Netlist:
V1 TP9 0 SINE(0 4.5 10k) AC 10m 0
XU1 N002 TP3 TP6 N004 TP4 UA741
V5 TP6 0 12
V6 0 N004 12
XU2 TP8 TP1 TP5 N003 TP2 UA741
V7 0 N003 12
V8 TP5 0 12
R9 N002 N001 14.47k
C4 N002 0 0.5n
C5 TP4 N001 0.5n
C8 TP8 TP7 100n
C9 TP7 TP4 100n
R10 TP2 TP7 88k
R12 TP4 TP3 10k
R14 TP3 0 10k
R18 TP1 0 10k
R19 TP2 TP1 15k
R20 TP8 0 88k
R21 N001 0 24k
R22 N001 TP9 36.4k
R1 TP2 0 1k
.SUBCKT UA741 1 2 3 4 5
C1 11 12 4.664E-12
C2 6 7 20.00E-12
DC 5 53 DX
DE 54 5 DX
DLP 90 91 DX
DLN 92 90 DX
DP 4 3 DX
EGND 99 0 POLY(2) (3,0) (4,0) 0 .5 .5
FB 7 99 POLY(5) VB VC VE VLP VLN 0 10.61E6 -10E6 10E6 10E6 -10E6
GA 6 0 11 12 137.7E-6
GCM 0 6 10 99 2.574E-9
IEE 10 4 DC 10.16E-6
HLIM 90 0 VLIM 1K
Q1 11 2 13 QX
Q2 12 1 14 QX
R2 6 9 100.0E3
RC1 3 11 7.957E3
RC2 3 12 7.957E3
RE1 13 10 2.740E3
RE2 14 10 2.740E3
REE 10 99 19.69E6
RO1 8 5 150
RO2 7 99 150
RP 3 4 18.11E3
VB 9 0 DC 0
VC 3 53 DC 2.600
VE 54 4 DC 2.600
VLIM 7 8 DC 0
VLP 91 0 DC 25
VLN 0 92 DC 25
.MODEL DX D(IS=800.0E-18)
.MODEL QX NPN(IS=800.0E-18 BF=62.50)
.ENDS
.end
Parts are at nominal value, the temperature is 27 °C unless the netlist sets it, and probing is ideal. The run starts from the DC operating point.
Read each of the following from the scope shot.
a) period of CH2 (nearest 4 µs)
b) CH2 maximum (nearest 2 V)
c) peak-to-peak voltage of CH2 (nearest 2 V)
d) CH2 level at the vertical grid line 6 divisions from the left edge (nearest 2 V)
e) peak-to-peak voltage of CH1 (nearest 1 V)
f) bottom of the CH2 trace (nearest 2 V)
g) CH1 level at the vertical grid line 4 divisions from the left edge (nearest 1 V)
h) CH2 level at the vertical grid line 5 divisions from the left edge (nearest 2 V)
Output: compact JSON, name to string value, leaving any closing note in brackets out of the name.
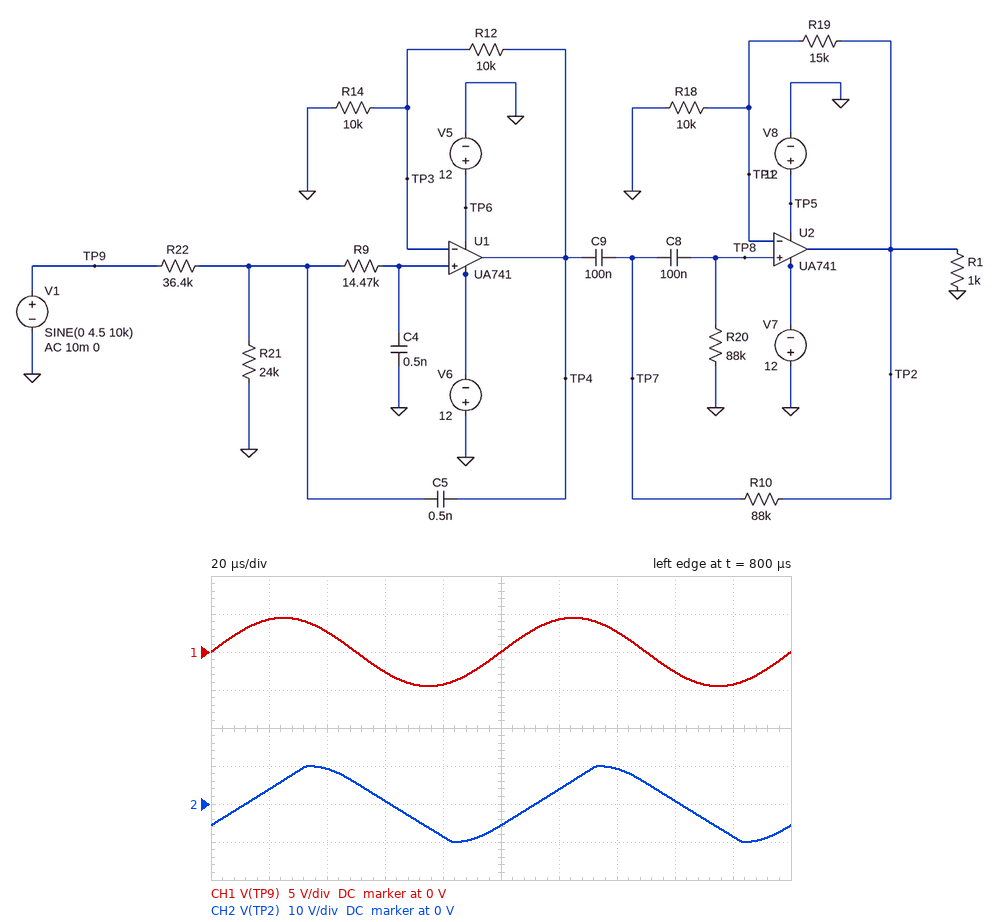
{"period of CH2": "100 µs", "CH2 maximum": "10 V", "peak-to-peak voltage of CH2": "20 V", "CH2 level at the vertical grid line 6 divisions from the left edge": "4 V", "peak-to-peak voltage of CH1": "9 V", "bottom of the CH2 trace": "-10 V", "CH1 level at the vertical grid line 4 divisions from the left edge": "-4 V", "CH2 level at the vertical grid line 5 divisions from the left edge": "-6 V"}
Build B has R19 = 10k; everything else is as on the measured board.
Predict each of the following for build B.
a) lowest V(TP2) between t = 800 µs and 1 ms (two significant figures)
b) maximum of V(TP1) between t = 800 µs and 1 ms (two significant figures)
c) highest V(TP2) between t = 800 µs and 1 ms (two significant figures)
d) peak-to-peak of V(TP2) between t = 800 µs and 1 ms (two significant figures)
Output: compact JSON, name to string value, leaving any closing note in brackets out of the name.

{"lowest V(TP2) between t = 800 µs and 1 ms": "-8.0 V", "maximum of V(TP1) between t = 800 µs and 1 ms": "4.0 V", "highest V(TP2) between t = 800 µs and 1 ms": "7.9 V", "peak-to-peak of V(TP2) between t = 800 µs and 1 ms": "16 V"}
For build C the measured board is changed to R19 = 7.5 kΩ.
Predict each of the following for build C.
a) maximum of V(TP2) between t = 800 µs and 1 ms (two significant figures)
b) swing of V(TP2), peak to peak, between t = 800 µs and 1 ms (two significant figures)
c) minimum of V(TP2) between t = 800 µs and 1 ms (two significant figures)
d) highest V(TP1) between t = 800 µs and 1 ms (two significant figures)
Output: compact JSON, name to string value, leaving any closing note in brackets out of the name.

{"maximum of V(TP2) between t = 800 µs and 1 ms": "6.9 V", "swing of V(TP2), peak to peak, between t = 800 µs and 1 ms": "14 V", "minimum of V(TP2) between t = 800 µs and 1 ms": "-7.0 V", "highest V(TP1) between t = 800 µs and 1 ms": "4.0 V"}
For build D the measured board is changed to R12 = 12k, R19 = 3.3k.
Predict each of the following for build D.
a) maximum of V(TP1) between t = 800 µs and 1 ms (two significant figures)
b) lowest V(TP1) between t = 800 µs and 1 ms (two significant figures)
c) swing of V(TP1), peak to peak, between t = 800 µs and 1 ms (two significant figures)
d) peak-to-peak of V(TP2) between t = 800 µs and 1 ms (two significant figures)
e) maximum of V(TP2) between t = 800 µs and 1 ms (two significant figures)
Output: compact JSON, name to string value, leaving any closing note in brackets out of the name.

{"maximum of V(TP1) between t = 800 µs and 1 ms": "4.6 V", "lowest V(TP1) between t = 800 µs and 1 ms": "-4.6 V", "swing of V(TP1), peak to peak, between t = 800 µs and 1 ms": "9.2 V", "peak-to-peak of V(TP2) between t = 800 µs and 1 ms": "12 V", "maximum of V(TP2) between t = 800 µs and 1 ms": "6.1 V"}
